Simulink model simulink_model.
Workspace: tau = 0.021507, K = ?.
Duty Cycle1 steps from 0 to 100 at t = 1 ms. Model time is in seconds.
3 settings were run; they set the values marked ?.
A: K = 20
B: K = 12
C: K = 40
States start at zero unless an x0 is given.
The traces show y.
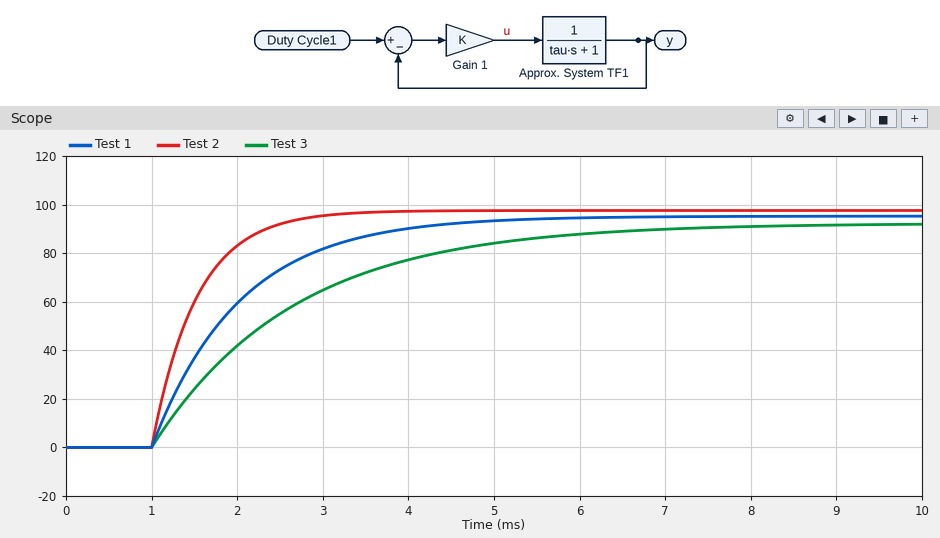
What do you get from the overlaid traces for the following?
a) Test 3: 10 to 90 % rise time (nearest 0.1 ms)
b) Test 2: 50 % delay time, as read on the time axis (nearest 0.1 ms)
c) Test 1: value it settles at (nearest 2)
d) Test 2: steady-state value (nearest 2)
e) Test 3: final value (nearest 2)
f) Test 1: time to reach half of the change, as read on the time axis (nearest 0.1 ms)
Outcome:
3.6 ms
1.4 ms
96
98
92
1.7 ms
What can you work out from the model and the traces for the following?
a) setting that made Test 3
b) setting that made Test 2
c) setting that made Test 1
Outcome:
B
C
A
